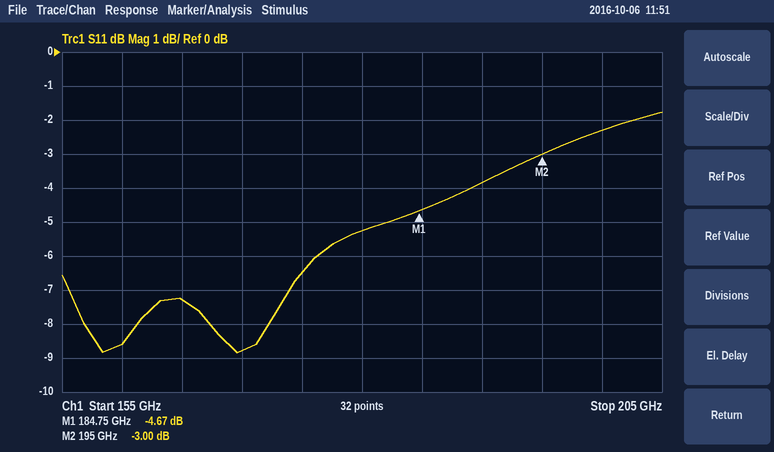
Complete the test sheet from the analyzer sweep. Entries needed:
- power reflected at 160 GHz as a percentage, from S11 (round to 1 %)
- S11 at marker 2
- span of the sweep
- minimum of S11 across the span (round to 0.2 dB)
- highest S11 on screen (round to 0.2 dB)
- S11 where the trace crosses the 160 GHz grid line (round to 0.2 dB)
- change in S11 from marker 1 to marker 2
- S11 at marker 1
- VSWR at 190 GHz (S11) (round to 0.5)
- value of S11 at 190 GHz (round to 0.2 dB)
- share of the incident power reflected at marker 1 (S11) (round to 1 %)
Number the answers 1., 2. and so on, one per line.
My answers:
1. 14 %
2. -3.00 dB
3. 50 GHz
4. -8.8 dB
5. -1.8 dB
6. -8.6 dB
7. 1.67 dB
8. -4.67 dB
9. 4.5
10. -3.8 dB
11. 34 %
